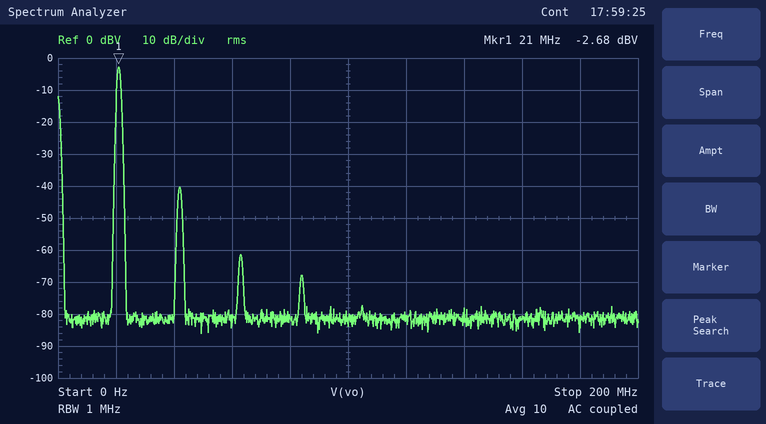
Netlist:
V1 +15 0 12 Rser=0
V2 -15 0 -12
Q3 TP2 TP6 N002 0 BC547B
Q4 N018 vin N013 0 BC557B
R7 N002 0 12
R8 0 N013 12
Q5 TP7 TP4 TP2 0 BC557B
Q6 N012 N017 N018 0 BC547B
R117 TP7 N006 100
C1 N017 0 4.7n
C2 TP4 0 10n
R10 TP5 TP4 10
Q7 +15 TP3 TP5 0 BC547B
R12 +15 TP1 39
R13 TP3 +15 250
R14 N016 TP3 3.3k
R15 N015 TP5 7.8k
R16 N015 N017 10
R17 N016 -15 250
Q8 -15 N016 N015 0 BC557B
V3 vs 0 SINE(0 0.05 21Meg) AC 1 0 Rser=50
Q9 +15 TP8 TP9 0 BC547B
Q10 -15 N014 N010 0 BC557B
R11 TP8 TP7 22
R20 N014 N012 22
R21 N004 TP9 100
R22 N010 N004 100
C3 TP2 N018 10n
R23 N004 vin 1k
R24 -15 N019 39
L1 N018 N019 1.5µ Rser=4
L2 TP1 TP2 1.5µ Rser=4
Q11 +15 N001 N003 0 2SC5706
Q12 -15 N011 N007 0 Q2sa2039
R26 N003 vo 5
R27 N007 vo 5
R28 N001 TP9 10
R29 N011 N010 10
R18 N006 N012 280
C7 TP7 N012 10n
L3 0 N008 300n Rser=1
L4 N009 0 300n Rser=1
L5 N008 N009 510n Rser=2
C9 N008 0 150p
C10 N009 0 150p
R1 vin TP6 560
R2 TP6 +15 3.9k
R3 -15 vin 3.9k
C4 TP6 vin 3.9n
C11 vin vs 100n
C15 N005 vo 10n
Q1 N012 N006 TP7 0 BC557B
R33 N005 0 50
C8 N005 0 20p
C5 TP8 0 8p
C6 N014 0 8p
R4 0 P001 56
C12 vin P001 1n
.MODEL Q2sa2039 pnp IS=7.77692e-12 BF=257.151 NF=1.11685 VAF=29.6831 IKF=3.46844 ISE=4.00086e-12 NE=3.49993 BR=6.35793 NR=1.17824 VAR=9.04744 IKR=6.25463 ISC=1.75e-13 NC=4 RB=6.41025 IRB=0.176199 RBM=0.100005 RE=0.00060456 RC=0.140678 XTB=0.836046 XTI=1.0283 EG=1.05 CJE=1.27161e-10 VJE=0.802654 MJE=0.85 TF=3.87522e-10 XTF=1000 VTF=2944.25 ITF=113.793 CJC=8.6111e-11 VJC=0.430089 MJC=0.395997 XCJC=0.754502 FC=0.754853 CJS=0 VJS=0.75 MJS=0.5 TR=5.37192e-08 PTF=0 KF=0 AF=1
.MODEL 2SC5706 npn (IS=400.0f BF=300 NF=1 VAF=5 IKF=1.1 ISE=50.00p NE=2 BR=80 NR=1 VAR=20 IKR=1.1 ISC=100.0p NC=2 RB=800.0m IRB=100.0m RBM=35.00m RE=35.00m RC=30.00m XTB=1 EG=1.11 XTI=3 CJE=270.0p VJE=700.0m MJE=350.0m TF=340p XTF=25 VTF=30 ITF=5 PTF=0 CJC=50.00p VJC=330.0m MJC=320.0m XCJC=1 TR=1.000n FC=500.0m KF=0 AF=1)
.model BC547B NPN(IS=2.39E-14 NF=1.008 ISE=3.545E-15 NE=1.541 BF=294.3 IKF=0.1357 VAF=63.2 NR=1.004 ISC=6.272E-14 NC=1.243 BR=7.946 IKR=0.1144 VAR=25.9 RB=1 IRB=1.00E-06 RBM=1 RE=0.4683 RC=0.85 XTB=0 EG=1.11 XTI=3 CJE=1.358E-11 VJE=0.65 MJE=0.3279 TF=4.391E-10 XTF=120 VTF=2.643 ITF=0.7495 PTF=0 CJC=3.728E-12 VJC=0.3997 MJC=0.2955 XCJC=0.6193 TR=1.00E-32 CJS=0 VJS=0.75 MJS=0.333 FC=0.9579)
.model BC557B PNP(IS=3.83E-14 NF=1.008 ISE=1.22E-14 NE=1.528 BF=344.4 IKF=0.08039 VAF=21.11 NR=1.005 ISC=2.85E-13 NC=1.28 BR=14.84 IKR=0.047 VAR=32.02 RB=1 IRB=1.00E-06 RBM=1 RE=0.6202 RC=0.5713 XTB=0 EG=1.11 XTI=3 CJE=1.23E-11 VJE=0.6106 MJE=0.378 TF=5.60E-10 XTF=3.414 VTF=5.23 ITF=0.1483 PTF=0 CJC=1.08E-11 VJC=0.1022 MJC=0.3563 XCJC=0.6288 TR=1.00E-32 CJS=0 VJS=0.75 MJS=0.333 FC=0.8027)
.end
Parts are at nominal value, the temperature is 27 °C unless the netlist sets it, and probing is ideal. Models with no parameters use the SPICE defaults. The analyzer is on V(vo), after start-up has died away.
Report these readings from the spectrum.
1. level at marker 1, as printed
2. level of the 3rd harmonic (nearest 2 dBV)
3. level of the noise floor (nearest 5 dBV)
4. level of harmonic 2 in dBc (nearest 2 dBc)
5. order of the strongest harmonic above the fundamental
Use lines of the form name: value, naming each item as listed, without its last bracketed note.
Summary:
level at marker 1, as printed: -2.68 dBV
level of the 3rd harmonic: -62 dBV
level of the noise floor: -80 dBV
level of harmonic 2 in dBc: -38 dBc
order of the strongest harmonic above the fundamental: 2
